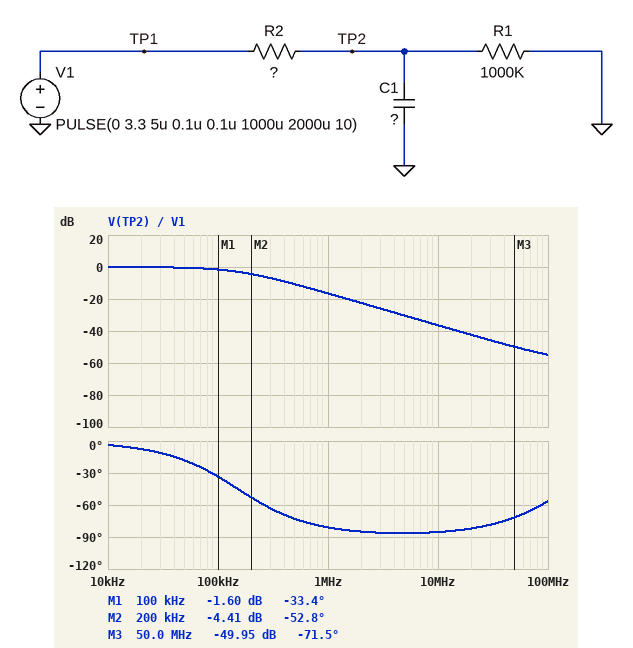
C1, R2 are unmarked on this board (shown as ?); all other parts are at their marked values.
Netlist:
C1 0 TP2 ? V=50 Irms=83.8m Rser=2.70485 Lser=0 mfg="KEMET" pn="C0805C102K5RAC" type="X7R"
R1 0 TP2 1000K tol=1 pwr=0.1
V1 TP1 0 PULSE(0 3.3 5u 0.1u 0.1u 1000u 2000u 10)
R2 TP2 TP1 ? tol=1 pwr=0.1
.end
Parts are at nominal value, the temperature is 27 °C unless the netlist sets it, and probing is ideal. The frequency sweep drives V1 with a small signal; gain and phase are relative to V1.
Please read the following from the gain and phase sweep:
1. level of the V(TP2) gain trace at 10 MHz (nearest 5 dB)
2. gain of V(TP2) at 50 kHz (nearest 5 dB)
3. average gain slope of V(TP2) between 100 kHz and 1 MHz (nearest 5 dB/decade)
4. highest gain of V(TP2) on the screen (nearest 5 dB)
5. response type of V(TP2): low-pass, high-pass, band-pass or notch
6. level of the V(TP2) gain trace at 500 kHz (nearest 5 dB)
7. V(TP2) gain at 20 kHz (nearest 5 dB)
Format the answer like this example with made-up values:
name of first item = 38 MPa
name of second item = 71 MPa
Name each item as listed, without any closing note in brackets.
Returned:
level of the V(TP2) gain trace at 10 MHz = -35 dB
gain of V(TP2) at 50 kHz = 0 dB
average gain slope of V(TP2) between 100 kHz and 1 MHz = -15 dB/decade
highest gain of V(TP2) on the screen = 0 dB
response type of V(TP2): low-pass, high-pass, band-pass or notch = low-pass
level of the V(TP2) gain trace at 500 kHz = -10 dB
V(TP2) gain at 20 kHz = 0 dB
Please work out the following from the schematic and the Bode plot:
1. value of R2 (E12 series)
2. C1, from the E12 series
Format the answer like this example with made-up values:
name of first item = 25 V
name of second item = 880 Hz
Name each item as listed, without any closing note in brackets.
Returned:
value of R2 = 2.7 kΩ
C1, from the E12 series = 390 pF
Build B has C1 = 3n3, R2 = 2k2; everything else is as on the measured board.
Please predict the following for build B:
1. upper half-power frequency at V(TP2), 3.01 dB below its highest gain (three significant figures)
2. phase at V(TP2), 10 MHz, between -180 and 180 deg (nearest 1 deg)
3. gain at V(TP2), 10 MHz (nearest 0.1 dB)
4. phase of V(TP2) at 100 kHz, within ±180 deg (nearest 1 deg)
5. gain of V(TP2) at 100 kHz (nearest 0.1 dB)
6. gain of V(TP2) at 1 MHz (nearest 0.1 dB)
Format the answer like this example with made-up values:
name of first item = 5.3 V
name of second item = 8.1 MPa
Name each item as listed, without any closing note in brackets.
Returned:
upper half-power frequency at V(TP2), 3.01 dB below its highest gain = 21.9 kHz
phase at V(TP2), 10 MHz, between -180 and 180 deg = -61 deg
gain at V(TP2), 10 MHz = -52.0 dB
phase of V(TP2) at 100 kHz, within ±180 deg = -77 deg
gain of V(TP2) at 100 kHz = -13.4 dB
gain of V(TP2) at 1 MHz = -33.2 dB
